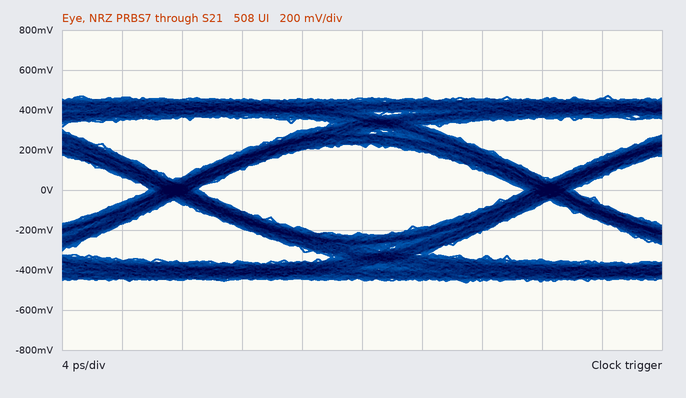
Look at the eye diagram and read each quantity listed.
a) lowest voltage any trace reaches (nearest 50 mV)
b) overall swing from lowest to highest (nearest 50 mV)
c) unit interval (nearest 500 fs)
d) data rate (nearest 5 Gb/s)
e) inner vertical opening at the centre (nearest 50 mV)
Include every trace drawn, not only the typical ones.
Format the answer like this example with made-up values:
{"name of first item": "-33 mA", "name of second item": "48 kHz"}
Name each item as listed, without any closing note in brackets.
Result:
{"lowest voltage any trace reaches": "-450 mV", "overall swing from lowest to highest": "950 mV", "unit interval": "25.0 ps", "data rate": "40 Gb/s", "inner vertical opening at the centre": "450 mV"}
